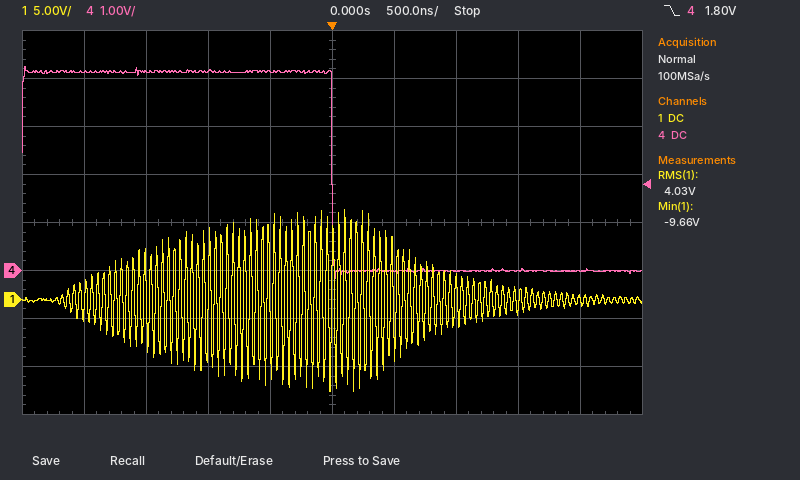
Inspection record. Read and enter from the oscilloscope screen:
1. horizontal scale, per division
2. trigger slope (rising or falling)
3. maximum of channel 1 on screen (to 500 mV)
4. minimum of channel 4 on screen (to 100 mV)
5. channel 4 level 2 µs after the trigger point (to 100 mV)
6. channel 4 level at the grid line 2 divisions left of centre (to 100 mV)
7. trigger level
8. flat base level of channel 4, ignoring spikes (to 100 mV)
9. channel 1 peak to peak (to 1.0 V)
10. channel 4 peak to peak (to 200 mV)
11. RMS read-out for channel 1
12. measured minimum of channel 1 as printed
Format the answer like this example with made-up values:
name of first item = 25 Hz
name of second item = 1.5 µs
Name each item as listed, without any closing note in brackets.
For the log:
horizontal scale, per division = 500 ns
trigger slope = falling
maximum of channel 1 on screen = 9.5 V
minimum of channel 4 on screen = -200 mV
channel 4 level 2 µs after the trigger point = 0.0 V
channel 4 level at the grid line 2 divisions left of centre = 4.2 V
trigger level = 1.80 V
flat base level of channel 4, ignoring spikes = 0.0 V
channel 1 peak to peak = 19.0 V
channel 4 peak to peak = 4.4 V
RMS read-out for channel 1 = 4.03 V
measured minimum of channel 1 as printed = -9.66 V
